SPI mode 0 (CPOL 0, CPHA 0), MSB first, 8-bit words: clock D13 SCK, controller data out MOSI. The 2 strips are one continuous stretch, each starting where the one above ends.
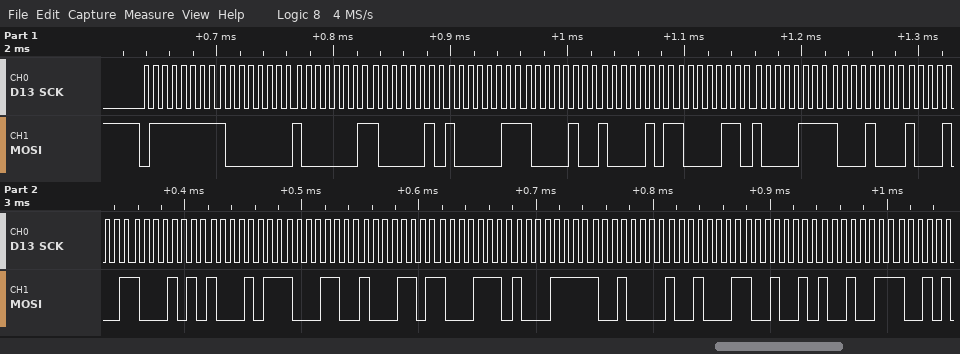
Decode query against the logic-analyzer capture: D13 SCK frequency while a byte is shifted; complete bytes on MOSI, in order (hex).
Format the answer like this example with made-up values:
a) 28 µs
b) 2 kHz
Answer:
a) 125 kHz
b) 7F 80 81 82 83 84 85 86 87 88 89 8A 8B 8C 8D 8E 8F 90 91 92 93
